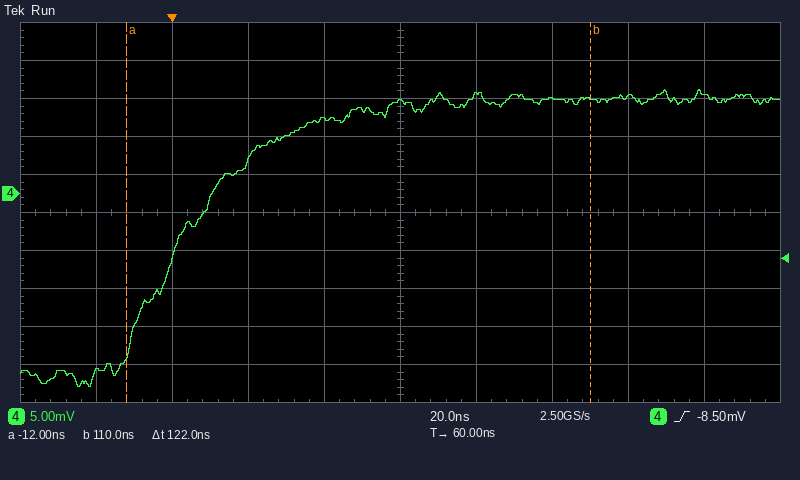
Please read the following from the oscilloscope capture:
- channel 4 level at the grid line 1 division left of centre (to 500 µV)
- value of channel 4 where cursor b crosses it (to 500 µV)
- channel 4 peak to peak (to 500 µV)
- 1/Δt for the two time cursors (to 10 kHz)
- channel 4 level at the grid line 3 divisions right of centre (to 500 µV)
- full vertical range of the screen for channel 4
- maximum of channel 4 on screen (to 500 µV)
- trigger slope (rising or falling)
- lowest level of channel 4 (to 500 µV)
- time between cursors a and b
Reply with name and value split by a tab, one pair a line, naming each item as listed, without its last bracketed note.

channel 4 level at the grid line 1 division left of centre	10.0 mV
value of channel 4 where cursor b crosses it	12.5 mV
channel 4 peak to peak	39.0 mV
1/Δt for the two time cursors	8.20 MHz
channel 4 level at the grid line 3 divisions right of centre	12.5 mV
full vertical range of the screen for channel 4	50 mV
maximum of channel 4 on screen	13.5 mV
trigger slope	rising
lowest level of channel 4	-25.5 mV
time between cursors a and b	122 ns
